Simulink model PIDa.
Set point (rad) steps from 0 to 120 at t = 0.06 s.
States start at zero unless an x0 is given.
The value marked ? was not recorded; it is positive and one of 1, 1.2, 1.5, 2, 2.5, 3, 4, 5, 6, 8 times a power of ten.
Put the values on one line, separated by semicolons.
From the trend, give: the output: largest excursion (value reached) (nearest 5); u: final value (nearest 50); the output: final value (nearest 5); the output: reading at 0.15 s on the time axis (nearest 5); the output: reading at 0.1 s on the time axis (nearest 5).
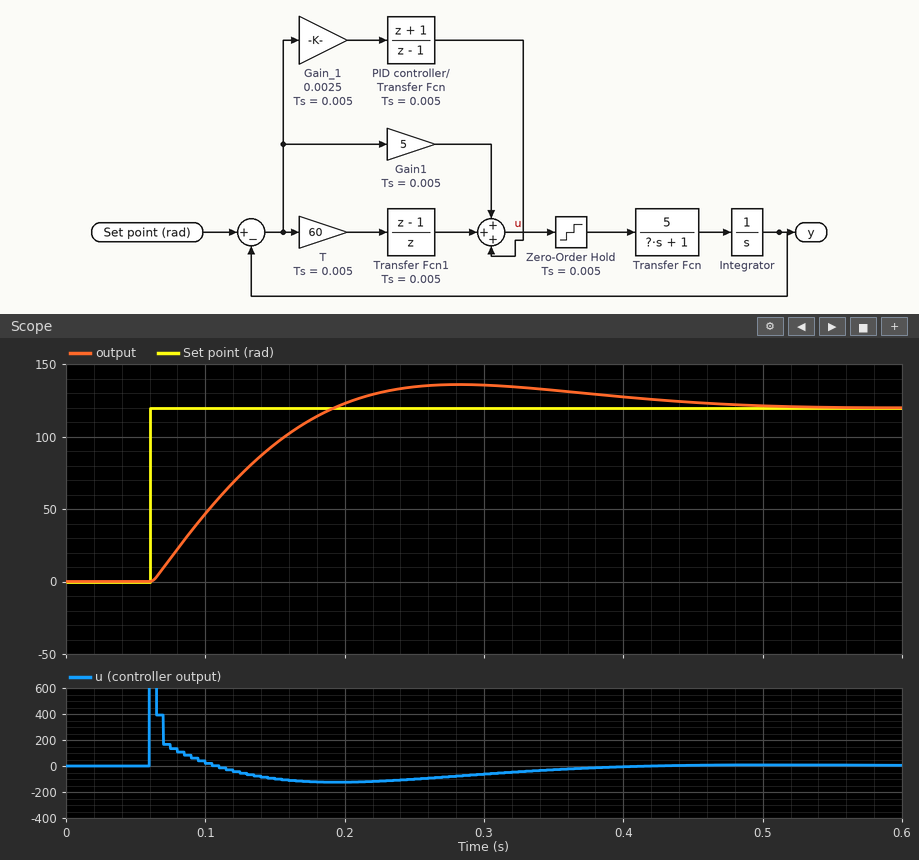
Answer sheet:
135; 0; 120; 95; 45
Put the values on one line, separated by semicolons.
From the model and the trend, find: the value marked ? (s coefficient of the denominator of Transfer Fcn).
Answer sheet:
0.15
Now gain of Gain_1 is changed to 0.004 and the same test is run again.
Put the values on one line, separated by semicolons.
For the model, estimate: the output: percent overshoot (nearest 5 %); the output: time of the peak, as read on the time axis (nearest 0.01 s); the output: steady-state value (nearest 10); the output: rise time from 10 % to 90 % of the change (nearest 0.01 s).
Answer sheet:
15 %; 0.28 s; 120; 0.10 s
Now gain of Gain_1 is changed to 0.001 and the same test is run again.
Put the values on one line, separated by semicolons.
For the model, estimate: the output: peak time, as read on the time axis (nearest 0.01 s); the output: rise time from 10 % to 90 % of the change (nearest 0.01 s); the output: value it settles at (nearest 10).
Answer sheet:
0.28 s; 0.10 s; 120
